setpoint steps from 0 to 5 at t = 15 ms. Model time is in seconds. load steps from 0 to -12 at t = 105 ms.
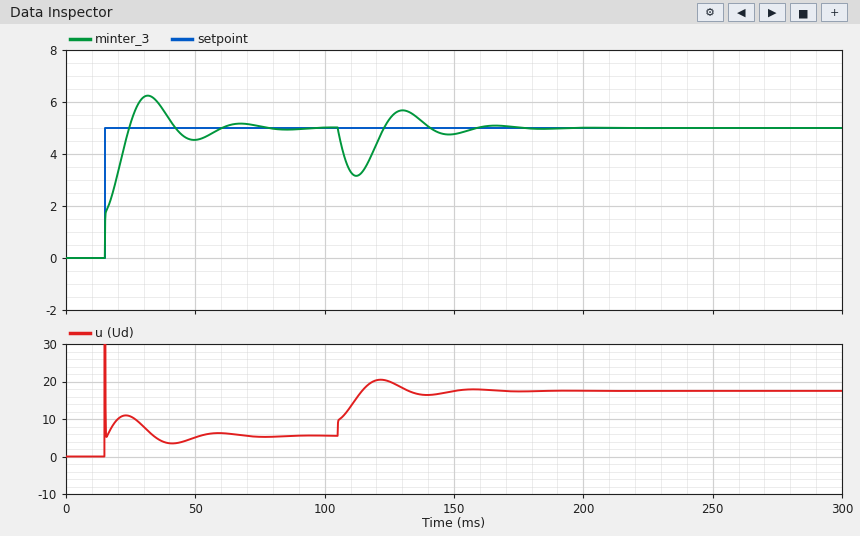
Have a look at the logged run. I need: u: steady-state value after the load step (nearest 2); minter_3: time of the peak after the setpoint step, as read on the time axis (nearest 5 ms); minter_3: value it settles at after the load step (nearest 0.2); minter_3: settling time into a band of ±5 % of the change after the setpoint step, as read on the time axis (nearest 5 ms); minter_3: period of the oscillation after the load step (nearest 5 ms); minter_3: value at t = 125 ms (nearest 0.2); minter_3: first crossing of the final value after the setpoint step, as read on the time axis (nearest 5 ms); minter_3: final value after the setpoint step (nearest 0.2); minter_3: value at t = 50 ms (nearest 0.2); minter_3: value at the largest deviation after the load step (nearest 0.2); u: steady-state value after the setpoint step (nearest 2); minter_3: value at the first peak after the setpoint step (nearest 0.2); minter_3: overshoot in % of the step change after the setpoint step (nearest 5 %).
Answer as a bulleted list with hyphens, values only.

- 18
- 30 ms
- 5.0
- 55 ms
- 35 ms
- 5.4
- 25 ms
- 5.0
- 4.6
- 3.2
- 6
- 6.2
- 25 %
